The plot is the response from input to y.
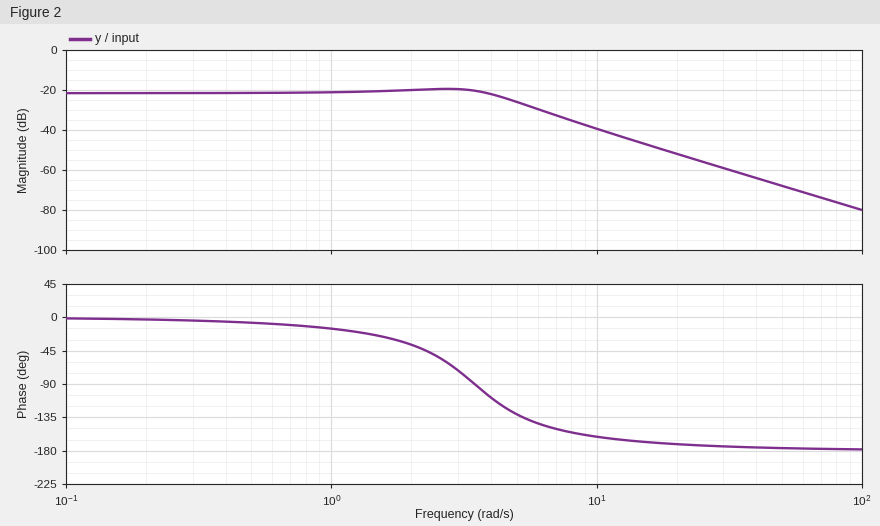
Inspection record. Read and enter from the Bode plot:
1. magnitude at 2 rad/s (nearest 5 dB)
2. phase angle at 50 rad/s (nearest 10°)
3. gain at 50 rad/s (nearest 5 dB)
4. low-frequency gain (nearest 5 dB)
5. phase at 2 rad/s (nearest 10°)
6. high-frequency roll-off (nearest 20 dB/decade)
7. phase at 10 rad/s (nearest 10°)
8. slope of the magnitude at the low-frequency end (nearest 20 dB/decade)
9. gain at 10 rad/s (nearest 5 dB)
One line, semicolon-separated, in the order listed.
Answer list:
-20 dB; -180°; -70 dB; -20 dB; -40°; -40 dB/decade; -160°; 0 dB/decade; -40 dB
